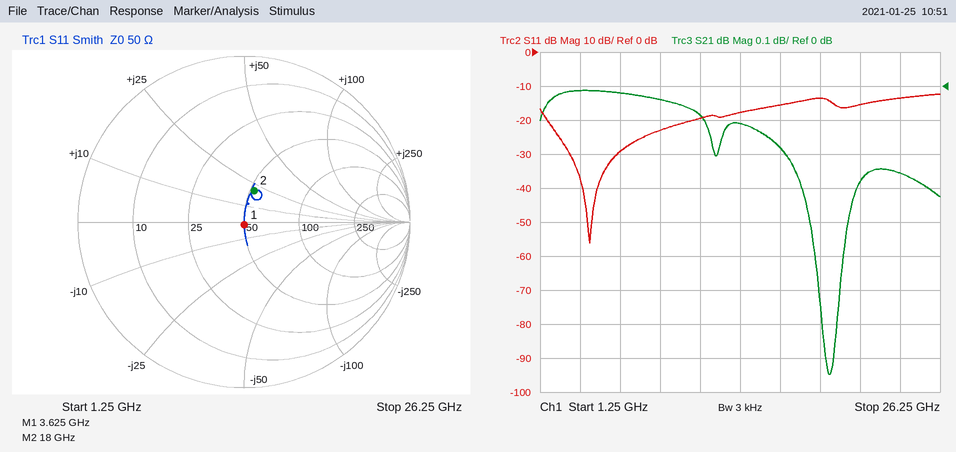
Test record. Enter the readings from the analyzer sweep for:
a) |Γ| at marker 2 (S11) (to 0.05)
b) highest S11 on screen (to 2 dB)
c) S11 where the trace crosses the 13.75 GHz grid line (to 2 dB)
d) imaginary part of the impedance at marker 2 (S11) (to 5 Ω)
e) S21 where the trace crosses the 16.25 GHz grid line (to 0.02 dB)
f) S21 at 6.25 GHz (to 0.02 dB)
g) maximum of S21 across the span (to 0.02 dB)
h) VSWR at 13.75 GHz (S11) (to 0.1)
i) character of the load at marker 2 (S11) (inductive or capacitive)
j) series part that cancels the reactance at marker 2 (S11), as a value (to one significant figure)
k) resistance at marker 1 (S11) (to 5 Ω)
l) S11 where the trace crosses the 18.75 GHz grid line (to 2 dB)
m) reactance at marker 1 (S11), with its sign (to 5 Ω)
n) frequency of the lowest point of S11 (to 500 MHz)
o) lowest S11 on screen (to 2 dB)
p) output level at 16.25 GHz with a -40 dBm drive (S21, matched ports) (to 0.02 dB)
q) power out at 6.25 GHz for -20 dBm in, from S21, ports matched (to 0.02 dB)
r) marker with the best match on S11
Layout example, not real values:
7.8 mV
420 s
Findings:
0.20
-12 dB
-18 dB
+20 Ω
-0.18 dB
-0.02 dB
-0.02 dB
1.3
inductive
400 fF
50 Ω
-14 dB
0 Ω
4.5 GHz
-56 dB
-40.18 dBm
-20.02 dBm
marker 1
